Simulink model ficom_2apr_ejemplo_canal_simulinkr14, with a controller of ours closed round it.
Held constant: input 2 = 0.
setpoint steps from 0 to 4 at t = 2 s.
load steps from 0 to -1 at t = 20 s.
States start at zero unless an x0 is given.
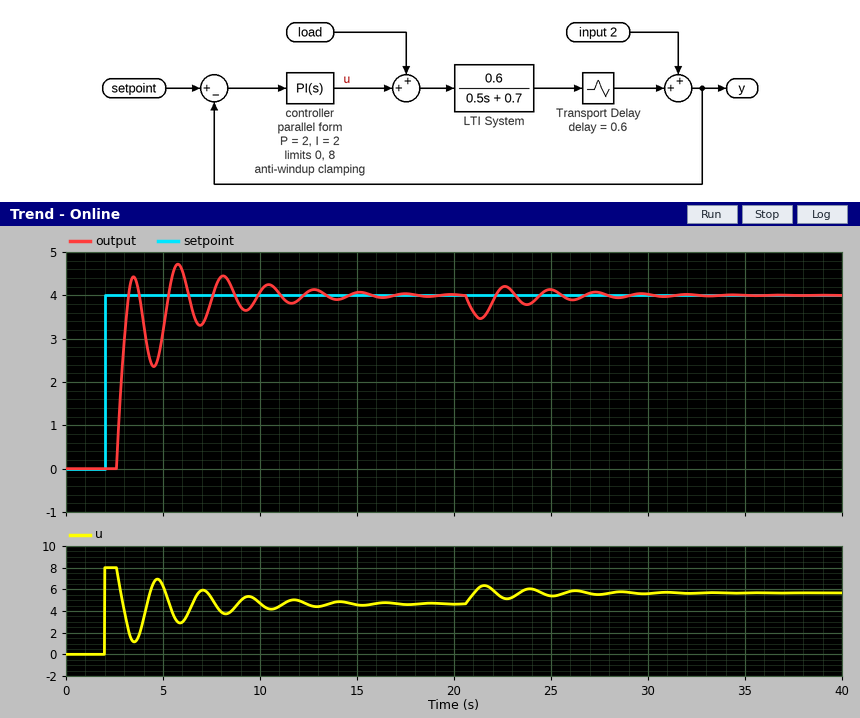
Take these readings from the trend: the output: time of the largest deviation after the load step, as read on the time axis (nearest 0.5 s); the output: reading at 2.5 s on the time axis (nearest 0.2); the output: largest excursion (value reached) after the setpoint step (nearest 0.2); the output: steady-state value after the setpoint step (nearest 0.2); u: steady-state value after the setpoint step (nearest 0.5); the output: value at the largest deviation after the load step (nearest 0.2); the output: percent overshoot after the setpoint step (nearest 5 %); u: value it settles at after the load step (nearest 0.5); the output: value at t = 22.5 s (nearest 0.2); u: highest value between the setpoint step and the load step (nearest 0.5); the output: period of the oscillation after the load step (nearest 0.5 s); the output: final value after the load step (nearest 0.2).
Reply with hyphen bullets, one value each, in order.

- 21.5 s
- 0.0
- 4.8
- 4.0
- 4.5
- 3.4
- 20 %
- 5.5
- 4.2
- 8.0
- 2.5 s
- 4.0
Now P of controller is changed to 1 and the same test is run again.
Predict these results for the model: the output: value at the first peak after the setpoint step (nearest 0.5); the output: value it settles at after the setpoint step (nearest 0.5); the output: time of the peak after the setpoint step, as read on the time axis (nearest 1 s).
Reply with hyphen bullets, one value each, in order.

- 5.5
- 4.0
- 4 s
